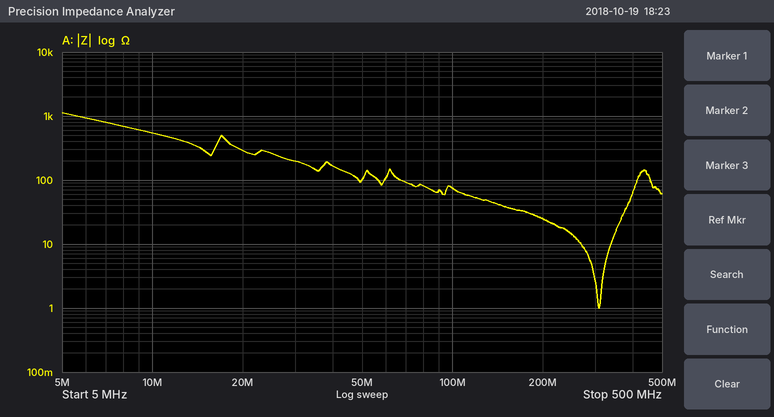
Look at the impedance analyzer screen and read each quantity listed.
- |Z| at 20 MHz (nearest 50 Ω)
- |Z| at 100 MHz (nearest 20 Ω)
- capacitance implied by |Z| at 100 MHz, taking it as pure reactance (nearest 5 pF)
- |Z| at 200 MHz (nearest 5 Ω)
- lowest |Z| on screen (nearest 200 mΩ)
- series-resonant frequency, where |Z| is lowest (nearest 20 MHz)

300 Ω
80 Ω
20 pF
25 Ω
1.0 Ω
300 MHz
